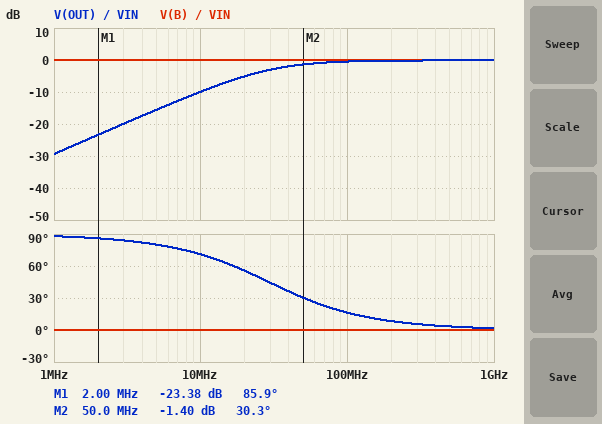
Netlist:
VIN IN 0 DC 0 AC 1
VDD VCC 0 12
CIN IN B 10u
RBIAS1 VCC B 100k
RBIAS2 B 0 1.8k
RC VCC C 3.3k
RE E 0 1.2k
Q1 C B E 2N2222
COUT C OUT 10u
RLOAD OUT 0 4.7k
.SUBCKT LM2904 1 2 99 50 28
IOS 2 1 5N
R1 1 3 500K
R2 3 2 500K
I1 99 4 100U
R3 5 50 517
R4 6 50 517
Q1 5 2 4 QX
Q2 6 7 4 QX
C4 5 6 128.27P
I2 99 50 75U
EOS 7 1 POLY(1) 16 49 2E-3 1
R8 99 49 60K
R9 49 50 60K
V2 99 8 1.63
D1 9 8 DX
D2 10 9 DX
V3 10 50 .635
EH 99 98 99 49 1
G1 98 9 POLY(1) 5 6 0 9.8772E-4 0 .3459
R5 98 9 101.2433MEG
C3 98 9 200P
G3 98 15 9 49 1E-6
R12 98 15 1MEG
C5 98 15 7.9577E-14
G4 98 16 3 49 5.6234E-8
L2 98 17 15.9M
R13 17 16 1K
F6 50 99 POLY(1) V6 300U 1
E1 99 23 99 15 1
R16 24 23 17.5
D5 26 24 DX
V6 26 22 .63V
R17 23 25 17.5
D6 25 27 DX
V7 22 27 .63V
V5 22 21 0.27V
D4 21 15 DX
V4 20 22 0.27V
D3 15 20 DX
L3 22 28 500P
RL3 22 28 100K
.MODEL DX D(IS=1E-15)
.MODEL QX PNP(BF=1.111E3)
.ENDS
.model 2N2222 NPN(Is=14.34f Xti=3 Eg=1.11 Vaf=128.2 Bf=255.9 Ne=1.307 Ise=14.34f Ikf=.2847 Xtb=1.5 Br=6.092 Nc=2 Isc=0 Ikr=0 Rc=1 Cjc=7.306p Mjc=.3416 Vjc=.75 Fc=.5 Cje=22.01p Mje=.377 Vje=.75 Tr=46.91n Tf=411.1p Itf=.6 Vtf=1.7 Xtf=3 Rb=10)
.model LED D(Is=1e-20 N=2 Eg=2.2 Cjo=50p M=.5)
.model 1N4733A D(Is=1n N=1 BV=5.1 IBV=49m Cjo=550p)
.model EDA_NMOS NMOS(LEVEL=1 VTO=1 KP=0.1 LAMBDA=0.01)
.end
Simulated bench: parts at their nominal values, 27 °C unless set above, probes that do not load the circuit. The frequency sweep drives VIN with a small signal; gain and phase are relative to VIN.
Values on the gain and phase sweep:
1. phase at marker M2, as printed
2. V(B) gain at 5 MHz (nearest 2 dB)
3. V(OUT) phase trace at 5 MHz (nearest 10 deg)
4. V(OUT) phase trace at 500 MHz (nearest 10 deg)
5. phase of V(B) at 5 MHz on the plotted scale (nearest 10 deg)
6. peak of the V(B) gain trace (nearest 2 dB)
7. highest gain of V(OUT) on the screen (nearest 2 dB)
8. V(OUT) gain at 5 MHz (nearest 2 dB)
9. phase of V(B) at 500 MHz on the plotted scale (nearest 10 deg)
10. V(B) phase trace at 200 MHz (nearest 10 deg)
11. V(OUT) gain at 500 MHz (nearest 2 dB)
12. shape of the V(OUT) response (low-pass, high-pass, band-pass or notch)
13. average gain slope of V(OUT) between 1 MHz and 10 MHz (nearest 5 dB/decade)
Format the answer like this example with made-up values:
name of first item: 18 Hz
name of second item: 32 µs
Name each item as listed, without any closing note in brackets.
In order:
phase at marker M2, as printed: 30.3 deg
V(B) gain at 5 MHz: 0 dB
V(OUT) phase trace at 5 MHz: 80 deg
V(OUT) phase trace at 500 MHz: 0 deg
phase of V(B) at 5 MHz on the plotted scale: 0 deg
peak of the V(B) gain trace: 0 dB
highest gain of V(OUT) on the screen: 0 dB
V(OUT) gain at 5 MHz: -16 dB
phase of V(B) at 500 MHz on the plotted scale: 0 deg
V(B) phase trace at 200 MHz: 0 deg
V(OUT) gain at 500 MHz: 0 dB
shape of the V(OUT) response: high-pass
average gain slope of V(OUT) between 1 MHz and 10 MHz: 20 dB/decade
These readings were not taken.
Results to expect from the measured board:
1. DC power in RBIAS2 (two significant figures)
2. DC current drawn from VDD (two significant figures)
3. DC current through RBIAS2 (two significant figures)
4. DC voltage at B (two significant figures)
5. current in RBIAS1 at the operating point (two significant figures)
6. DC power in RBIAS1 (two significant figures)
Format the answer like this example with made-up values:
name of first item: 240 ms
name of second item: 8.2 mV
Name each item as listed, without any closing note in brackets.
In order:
DC power in RBIAS2: 25 µW
DC current drawn from VDD: 120 µA
DC current through RBIAS2: 120 µA
DC voltage at B: 210 mV
current in RBIAS1 at the operating point: 120 µA
DC power in RBIAS1: 1.4 mW
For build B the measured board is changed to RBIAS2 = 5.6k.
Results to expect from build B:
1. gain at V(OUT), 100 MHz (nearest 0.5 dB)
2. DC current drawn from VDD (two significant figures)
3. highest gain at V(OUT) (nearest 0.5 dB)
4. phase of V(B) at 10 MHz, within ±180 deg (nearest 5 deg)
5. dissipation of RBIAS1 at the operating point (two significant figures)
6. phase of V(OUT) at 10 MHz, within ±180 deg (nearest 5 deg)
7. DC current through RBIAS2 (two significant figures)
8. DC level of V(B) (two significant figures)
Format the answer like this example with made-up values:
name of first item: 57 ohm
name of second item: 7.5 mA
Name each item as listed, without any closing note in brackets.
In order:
gain at V(OUT), 100 MHz: 0 dB
DC current drawn from VDD: 170 µA
highest gain at V(OUT): 1.0 dB
phase of V(B) at 10 MHz, within ±180 deg: 0 deg
dissipation of RBIAS1 at the operating point: 1.3 mW
phase of V(OUT) at 10 MHz, within ±180 deg: 110 deg
DC current through RBIAS2: 110 µA
DC level of V(B): 630 mV
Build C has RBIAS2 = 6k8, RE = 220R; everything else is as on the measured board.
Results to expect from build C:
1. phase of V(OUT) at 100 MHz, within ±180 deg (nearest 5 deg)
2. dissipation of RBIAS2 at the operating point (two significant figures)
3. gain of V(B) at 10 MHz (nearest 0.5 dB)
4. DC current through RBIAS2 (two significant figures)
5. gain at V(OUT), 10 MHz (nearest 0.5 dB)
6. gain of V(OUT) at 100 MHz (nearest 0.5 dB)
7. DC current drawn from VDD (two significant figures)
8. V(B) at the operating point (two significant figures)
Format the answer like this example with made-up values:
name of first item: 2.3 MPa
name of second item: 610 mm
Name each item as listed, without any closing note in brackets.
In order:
phase of V(OUT) at 100 MHz, within ±180 deg: 40 deg
dissipation of RBIAS2 at the operating point: 81 µW
gain of V(B) at 10 MHz: 0 dB
DC current through RBIAS2: 110 µA
gain at V(OUT), 10 MHz: 16.5 dB
gain of V(OUT) at 100 MHz: 6.0 dB
DC current drawn from VDD: 630 µA
V(B) at the operating point: 740 mV
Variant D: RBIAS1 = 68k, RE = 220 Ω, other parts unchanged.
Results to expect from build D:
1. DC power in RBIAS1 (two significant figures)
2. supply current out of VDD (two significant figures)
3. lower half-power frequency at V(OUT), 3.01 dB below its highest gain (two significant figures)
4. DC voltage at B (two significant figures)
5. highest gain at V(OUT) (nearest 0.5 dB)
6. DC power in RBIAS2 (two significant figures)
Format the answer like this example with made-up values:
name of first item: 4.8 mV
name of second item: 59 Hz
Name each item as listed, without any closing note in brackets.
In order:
DC power in RBIAS1: 2.0 mW
supply current out of VDD: 170 µA
lower half-power frequency at V(OUT), 3.01 dB below its highest gain: 28 MHz
DC voltage at B: 310 mV
highest gain at V(OUT): -0.5 dB
DC power in RBIAS2: 53 µW
